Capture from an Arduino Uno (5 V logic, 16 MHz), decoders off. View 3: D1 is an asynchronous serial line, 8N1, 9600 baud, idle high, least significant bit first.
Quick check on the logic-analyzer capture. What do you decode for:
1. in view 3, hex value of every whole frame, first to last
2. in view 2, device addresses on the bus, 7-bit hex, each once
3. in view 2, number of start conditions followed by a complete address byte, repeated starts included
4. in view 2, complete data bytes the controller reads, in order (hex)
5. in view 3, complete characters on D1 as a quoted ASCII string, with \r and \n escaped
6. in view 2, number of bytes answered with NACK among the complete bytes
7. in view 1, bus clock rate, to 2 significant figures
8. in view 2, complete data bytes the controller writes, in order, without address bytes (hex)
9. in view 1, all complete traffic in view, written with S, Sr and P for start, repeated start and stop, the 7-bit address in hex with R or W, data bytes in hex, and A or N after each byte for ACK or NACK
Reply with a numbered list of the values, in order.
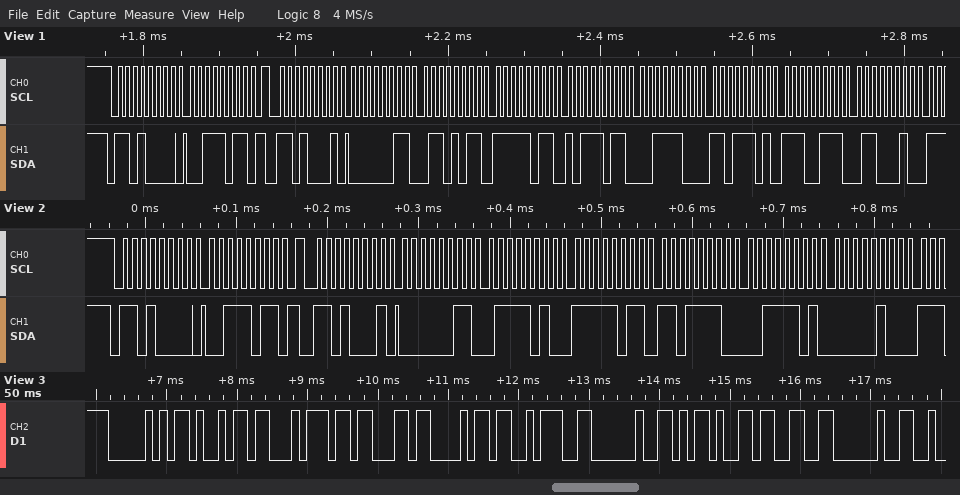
1. 0x50 0x69 0x74 0x63 0x68 0x3A 0x20 0x2D 0x33 0x20
2. 0x68
3. 2
4. 03 7A FB DE 3D 04
5. "Pitch: -3 "
6. 0
7. 100 kHz
8. 3B
9. S 68W A 3B A Sr 68R A 03 A 6B A FB A BB A 3C A DD A E7 A 62 A
